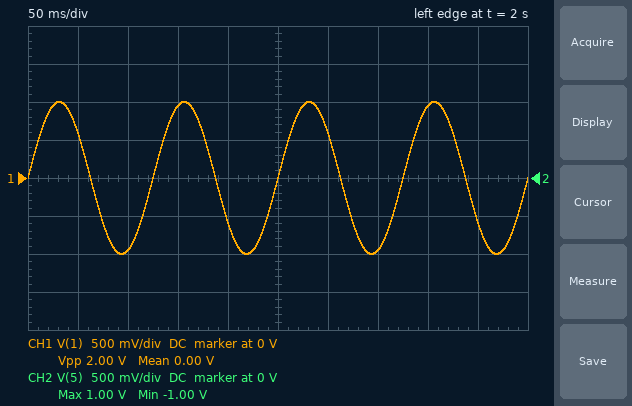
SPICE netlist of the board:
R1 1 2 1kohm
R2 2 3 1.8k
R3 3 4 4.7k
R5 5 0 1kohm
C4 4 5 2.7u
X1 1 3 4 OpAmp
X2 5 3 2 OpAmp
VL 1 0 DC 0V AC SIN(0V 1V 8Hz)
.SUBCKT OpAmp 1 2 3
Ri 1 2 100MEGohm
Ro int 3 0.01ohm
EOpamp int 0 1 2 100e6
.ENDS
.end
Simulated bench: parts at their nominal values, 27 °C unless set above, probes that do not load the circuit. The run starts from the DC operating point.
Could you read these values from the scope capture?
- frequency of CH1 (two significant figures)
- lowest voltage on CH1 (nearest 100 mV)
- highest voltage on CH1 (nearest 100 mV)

8.0 Hz
-1.0 V
1.0 V
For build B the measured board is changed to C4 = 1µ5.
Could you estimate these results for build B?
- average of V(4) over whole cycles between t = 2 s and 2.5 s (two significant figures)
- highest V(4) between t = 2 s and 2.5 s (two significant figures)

13 V
27 V
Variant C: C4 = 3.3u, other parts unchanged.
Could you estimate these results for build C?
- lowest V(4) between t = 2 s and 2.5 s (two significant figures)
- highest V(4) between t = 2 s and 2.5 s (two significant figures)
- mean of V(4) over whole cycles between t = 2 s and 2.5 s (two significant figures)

-82 mV
12 V
6.0 V
